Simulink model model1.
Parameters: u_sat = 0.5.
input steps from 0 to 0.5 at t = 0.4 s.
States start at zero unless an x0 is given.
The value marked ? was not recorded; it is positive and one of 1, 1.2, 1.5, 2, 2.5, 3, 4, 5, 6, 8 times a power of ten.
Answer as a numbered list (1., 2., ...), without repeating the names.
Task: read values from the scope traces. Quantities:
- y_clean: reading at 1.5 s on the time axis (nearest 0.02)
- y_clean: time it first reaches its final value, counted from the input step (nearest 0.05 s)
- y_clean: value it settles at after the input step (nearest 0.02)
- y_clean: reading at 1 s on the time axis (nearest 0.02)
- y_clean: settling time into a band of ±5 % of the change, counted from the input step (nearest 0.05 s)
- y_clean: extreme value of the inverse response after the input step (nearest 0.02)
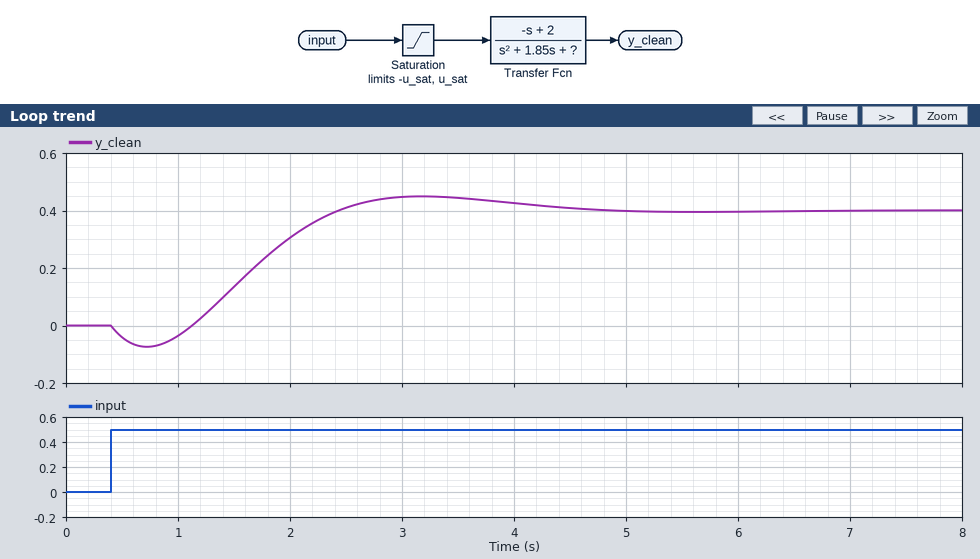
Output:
1. 0.14
2. 2.05 s
3. 0.40
4. -0.04
5. 3.75 s
6. -0.08
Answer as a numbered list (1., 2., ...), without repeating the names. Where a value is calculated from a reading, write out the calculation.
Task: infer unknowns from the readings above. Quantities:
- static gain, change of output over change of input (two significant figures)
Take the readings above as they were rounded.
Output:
1. (0.4 - 0) / (0.5 - 0) = 0.80
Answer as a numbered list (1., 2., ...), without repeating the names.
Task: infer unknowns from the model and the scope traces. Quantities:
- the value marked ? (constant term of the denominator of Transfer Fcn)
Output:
1. 2.5
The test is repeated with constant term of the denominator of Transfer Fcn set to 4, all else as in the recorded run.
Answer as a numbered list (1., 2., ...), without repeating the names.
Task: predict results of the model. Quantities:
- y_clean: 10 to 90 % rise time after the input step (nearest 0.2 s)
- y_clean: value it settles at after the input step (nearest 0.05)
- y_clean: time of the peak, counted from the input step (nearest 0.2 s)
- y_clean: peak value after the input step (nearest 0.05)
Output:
1. 0.6 s
2. 0.25
3. 2.0 s
4. 0.30
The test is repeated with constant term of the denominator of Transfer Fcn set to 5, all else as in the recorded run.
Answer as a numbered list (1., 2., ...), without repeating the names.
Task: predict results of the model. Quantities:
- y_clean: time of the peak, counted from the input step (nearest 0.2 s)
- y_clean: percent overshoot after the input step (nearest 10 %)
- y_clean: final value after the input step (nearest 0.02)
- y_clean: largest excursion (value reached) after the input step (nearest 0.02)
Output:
1. 1.8 s
2. 30 %
3. 0.20
4. 0.26
